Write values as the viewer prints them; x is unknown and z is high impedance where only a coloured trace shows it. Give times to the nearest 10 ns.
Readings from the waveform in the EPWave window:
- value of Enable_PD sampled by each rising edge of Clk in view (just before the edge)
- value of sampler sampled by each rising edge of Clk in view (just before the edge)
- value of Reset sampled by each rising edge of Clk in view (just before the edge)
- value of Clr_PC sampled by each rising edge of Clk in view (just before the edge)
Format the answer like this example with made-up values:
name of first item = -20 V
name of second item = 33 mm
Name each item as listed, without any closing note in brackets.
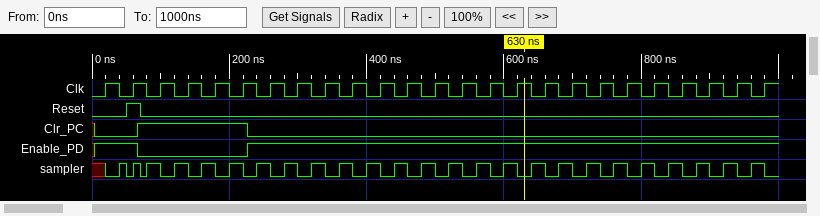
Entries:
value of Enable_PD sampled by each rising edge of Clk in view = 1 1 0 0 0 0 1 1 1 1 1 1 1 1 1 1 1 1 1 1 1 1 1 1 1
value of sampler sampled by each rising edge of Clk in view = x 0 1 1 1 1 1 1 1 1 1 1 1 1 1 1 1 1 1 1 1 1 1 1 1
value of Reset sampled by each rising edge of Clk in view = 0 1 0 0 0 0 0 0 0 0 0 0 0 0 0 0 0 0 0 0 0 0 0 0 0
value of Clr_PC sampled by each rising edge of Clk in view = 0 0 1 1 1 1 0 0 0 0 0 0 0 0 0 0 0 0 0 0 0 0 0 0 0
